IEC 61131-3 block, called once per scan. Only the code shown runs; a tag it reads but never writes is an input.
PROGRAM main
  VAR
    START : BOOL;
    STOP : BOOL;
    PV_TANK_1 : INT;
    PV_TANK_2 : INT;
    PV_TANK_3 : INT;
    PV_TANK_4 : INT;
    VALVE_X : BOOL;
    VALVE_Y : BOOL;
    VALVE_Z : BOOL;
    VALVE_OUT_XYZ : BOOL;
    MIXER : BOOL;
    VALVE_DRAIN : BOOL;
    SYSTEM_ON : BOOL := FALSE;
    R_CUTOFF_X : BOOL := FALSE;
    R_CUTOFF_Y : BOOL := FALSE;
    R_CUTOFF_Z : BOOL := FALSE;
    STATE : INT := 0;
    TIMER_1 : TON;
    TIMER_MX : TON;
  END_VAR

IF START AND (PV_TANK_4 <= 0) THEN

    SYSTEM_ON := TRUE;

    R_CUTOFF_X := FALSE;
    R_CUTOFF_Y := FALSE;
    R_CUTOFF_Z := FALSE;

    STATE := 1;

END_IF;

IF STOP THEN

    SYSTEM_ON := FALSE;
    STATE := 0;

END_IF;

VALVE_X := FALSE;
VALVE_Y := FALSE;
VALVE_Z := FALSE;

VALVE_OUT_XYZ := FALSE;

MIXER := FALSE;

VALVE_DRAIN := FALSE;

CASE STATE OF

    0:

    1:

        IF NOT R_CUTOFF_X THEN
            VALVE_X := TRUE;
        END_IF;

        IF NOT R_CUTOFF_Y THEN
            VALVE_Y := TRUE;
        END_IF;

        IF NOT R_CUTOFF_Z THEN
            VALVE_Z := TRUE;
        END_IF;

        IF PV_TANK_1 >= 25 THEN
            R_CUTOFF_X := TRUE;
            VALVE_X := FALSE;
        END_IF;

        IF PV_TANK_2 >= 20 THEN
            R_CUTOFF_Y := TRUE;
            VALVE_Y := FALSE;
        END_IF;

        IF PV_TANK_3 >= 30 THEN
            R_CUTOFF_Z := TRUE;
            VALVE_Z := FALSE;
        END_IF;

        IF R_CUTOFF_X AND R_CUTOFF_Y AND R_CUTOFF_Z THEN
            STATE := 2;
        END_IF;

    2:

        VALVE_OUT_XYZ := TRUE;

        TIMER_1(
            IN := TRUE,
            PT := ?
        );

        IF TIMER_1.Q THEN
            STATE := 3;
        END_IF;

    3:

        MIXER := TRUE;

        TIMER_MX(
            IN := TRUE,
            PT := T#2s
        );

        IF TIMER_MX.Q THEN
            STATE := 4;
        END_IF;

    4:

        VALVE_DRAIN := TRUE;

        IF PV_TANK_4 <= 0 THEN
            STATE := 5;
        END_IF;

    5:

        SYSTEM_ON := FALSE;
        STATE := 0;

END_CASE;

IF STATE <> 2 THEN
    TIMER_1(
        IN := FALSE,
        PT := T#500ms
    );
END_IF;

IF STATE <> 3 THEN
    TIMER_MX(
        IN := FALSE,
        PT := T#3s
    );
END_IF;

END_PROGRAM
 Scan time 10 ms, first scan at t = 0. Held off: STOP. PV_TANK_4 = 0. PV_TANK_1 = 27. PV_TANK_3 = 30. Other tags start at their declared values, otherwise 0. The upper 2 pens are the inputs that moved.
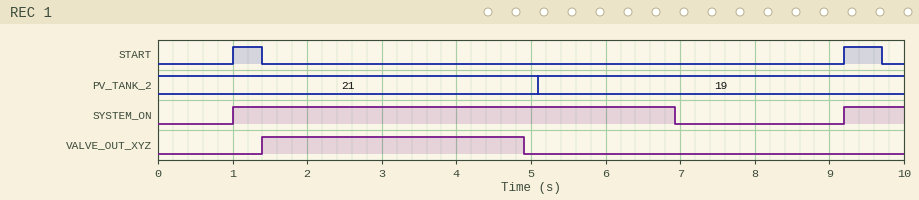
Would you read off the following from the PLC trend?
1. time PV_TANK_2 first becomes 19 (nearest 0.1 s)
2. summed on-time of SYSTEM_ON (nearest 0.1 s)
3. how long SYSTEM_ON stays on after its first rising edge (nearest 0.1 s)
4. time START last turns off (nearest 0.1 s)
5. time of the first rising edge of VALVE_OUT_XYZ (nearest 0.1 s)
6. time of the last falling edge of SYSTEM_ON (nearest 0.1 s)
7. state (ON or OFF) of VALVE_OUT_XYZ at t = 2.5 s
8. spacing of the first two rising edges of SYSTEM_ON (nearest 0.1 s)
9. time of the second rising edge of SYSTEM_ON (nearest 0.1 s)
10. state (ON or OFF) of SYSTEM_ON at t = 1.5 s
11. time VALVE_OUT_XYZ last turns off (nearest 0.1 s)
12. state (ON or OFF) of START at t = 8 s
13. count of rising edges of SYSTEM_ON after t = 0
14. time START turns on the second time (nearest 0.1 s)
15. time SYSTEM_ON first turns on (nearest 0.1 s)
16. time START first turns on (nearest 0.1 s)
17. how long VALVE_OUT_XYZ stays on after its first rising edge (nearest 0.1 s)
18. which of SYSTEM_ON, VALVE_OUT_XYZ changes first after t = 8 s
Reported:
5.1 s
6.7 s
5.9 s
9.7 s
1.4 s
6.9 s
ON
8.2 s
9.2 s
ON
4.9 s
OFF
2
9.2 s
1.0 s
1.0 s
3.5 s
SYSTEM_ON
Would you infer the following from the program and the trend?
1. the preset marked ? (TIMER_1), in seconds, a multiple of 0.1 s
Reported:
3.5 s
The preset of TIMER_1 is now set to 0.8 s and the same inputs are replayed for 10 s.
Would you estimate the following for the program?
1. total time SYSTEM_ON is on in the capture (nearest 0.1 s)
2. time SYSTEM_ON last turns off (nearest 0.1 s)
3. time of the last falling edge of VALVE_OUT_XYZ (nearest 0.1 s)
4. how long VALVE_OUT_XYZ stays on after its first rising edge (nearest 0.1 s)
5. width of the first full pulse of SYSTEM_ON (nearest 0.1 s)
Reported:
4.0 s
4.2 s
2.2 s
0.8 s
3.2 s
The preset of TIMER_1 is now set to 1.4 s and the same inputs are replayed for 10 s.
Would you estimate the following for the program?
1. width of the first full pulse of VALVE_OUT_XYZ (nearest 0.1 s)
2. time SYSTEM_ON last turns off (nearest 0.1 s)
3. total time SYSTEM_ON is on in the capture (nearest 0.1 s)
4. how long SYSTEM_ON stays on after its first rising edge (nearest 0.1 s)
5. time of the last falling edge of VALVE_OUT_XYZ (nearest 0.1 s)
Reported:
1.4 s
4.8 s
4.6 s
3.8 s
2.8 s
